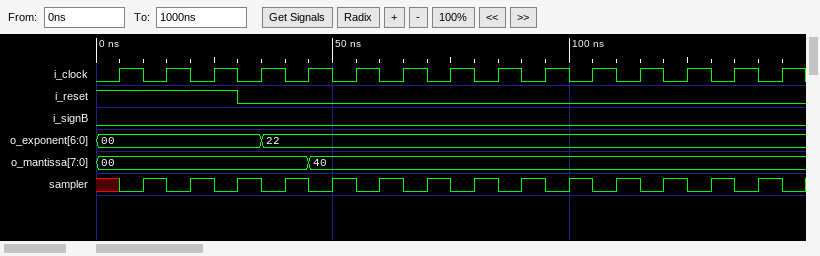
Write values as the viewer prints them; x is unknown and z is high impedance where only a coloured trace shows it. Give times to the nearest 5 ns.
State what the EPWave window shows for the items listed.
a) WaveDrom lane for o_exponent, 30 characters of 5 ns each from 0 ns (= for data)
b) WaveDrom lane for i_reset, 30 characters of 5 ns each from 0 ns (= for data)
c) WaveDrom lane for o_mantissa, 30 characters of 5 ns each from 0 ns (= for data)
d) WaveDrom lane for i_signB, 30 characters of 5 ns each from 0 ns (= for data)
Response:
{name: 'o_exponent', wave: '=......=......................', data: '00 22'}
{name: 'i_reset', wave: '1.....0.......................'}
{name: 'o_mantissa', wave: '=........=....................', data: '00 40'}
{name: 'i_signB', wave: '0.............................'}
